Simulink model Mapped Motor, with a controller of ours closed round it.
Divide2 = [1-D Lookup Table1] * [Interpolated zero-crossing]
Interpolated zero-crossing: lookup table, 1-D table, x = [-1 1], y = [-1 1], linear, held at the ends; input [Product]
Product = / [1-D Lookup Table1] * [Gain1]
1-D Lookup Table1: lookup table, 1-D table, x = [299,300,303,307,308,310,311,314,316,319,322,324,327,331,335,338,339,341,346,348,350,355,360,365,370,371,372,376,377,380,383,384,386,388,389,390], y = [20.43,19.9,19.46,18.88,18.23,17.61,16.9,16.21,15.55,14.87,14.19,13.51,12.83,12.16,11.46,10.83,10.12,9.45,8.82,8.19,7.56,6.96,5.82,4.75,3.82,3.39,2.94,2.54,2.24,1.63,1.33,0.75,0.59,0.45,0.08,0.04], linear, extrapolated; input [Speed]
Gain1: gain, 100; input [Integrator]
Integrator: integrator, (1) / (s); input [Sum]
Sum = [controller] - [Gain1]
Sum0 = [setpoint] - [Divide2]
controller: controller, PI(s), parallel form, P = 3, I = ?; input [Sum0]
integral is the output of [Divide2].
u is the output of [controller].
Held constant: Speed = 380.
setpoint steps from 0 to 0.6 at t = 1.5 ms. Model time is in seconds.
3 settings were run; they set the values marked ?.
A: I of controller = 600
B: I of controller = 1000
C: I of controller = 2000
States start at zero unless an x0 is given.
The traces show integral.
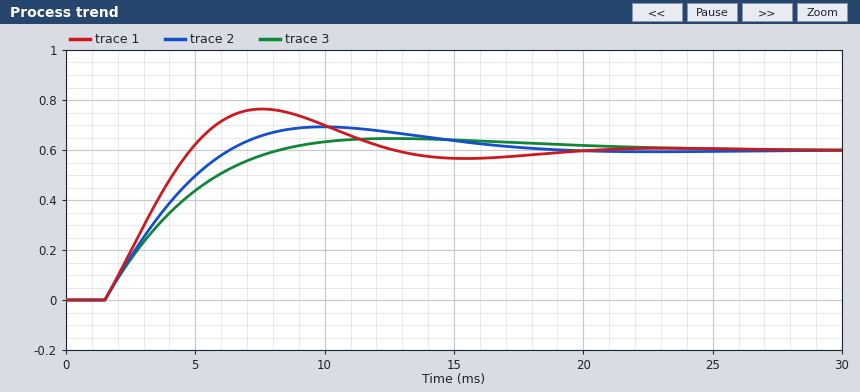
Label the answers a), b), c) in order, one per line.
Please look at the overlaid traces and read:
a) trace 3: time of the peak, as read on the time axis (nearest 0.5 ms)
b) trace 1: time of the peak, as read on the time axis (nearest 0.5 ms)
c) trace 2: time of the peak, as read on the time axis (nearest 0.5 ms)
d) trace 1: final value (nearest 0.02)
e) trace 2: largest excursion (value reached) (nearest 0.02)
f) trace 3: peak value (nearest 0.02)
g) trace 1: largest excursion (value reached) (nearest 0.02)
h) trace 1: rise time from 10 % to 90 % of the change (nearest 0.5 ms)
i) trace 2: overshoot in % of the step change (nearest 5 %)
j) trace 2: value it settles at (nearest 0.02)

a) 12.5 ms
b) 7.5 ms
c) 10.0 ms
d) 0.60
e) 0.70
f) 0.64
g) 0.76
h) 2.5 ms
i) 15 %
j) 0.60
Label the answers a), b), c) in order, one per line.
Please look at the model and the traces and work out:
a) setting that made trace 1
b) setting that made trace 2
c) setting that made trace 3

a) C
b) B
c) A
